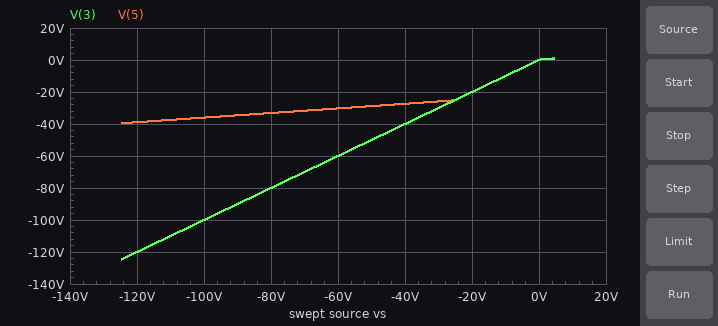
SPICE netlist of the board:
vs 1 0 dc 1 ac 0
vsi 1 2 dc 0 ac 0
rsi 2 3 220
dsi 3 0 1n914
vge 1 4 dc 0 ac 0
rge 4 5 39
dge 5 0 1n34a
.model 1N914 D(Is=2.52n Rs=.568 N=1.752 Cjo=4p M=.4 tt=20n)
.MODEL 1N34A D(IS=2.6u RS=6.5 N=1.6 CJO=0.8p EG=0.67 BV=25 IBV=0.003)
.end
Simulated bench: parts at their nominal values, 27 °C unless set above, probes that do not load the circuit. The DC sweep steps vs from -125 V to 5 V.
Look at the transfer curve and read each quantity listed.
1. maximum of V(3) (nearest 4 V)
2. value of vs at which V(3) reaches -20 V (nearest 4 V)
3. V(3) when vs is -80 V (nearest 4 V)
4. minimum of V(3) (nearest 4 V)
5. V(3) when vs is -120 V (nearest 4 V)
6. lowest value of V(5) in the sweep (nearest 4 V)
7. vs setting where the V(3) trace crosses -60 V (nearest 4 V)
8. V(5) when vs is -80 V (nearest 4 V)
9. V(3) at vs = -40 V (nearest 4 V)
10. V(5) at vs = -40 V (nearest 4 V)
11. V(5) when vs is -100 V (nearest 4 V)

0 V
-20 V
-80 V
-124 V
-120 V
-40 V
-60 V
-32 V
-40 V
-28 V
-36 V
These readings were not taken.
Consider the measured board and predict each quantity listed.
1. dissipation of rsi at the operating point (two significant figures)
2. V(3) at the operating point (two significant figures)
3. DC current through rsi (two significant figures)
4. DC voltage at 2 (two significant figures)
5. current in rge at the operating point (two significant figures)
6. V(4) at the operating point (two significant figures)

690 µW
610 mV
1.8 mA
1.0 V
14 mA
1.0 V
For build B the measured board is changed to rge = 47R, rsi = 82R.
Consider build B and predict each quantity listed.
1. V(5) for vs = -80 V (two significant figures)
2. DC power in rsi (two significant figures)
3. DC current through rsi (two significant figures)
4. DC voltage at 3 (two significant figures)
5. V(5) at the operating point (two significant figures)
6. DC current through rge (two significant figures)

-32 V
1.5 mW
4.2 mA
650 mV
430 mV
12 mA
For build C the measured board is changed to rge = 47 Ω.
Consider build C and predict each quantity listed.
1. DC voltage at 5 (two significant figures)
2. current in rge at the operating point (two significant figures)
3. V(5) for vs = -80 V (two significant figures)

430 mV
12 mA
-32 V
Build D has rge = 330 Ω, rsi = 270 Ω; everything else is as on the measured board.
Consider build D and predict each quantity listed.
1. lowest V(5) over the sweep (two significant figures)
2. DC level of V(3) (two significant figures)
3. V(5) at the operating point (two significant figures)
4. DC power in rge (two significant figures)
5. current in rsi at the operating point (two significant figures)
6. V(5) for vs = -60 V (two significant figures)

-27 V
600 mV
290 mV
1.5 mW
1.5 mA
-26 V
